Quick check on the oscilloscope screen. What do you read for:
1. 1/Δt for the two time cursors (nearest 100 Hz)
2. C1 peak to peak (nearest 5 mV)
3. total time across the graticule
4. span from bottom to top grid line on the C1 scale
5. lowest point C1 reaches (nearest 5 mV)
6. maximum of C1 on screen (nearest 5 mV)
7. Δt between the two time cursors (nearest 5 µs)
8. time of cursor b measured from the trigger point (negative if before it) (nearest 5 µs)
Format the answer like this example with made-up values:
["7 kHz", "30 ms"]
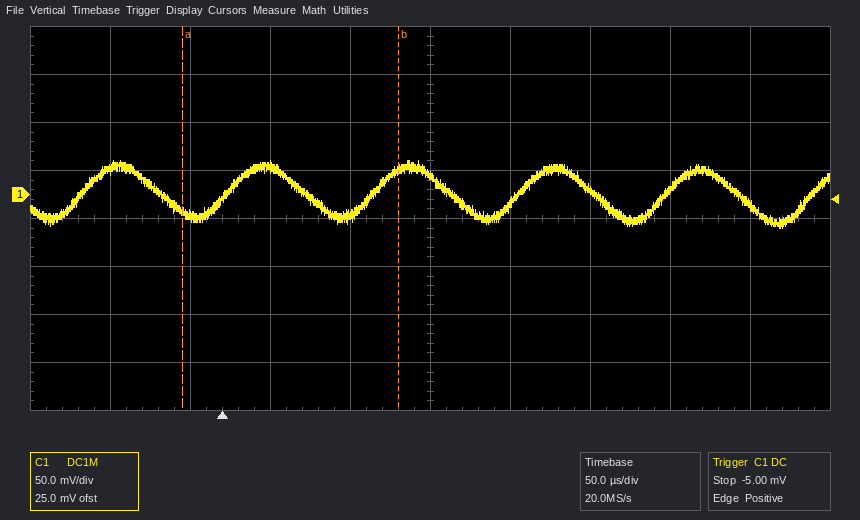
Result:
["7.4 kHz", "70 mV", "500 µs", "400 mV", "-35 mV", "35 mV", "135 µs", "+110 µs"]
